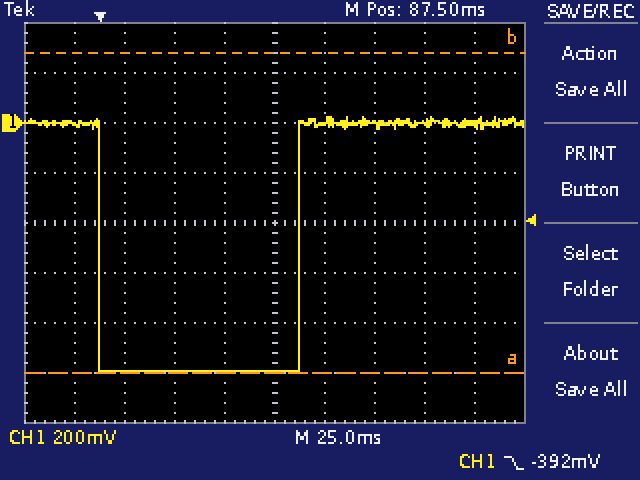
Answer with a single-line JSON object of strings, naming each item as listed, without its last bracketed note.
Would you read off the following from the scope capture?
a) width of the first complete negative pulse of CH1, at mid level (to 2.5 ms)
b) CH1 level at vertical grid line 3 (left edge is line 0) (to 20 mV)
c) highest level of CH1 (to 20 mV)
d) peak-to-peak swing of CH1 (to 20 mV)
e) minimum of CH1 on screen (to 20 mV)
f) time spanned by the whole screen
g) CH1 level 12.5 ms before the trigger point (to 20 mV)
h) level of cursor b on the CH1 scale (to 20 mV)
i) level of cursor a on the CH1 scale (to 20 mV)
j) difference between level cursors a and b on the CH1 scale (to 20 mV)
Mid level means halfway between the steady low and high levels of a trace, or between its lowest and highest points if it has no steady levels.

{"width of the first complete negative pulse of CH1, at mid level": "100.0 ms", "CH1 level at vertical grid line 3 (left edge is line 0)": "-1.00 V", "highest level of CH1": "20 mV", "peak-to-peak swing of CH1": "1.02 V", "minimum of CH1 on screen": "-1.00 V", "time spanned by the whole screen": "250 ms", "CH1 level 12.5 ms before the trigger point": "0 mV", "level of cursor b on the CH1 scale": "280 mV", "level of cursor a on the CH1 scale": "-1.00 V", "difference between level cursors a and b on the CH1 scale": "1.28 V"}
